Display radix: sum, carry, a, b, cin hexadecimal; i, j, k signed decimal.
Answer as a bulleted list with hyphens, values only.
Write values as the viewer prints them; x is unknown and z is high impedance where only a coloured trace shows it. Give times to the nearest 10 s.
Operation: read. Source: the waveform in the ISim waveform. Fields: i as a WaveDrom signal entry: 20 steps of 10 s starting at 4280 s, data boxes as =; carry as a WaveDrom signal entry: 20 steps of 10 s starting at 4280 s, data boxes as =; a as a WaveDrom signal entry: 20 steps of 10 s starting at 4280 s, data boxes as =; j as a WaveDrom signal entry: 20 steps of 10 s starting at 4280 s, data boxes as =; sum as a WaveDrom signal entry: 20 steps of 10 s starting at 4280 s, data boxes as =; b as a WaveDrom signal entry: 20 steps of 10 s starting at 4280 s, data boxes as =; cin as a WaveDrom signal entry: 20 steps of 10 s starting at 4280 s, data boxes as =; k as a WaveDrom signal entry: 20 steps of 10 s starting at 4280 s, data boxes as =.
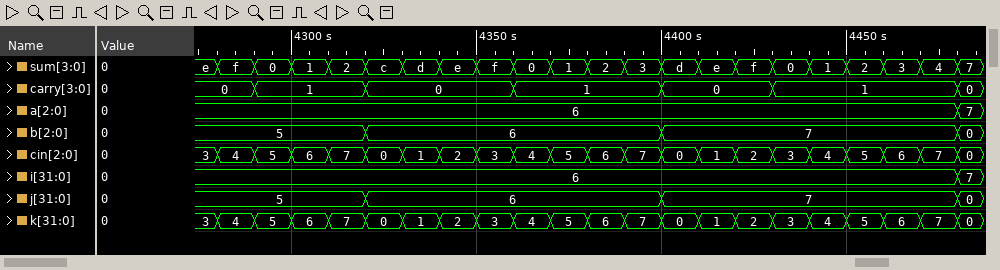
- {name: 'i', wave: '=...................', data: '6'}
- {name: 'carry', wave: '==..=...=...=..=....', data: '0 1 0 1 0 1'}
- {name: 'a', wave: '=...................', data: '6'}
- {name: 'j', wave: '=...=.......=.......', data: '5 6 7'}
- {name: 'sum', wave: '====================', data: 'f 0 1 2 c d e f 0 1 2 3 d e f 0 1 2 3 4'}
- {name: 'b', wave: '=...=.......=.......', data: '5 6 7'}
- {name: 'cin', wave: '====================', data: '4 5 6 7 0 1 2 3 4 5 6 7 0 1 2 3 4 5 6 7'}
- {name: 'k', wave: '====================', data: '4 5 6 7 0 1 2 3 4 5 6 7 0 1 2 3 4 5 6 7'}
